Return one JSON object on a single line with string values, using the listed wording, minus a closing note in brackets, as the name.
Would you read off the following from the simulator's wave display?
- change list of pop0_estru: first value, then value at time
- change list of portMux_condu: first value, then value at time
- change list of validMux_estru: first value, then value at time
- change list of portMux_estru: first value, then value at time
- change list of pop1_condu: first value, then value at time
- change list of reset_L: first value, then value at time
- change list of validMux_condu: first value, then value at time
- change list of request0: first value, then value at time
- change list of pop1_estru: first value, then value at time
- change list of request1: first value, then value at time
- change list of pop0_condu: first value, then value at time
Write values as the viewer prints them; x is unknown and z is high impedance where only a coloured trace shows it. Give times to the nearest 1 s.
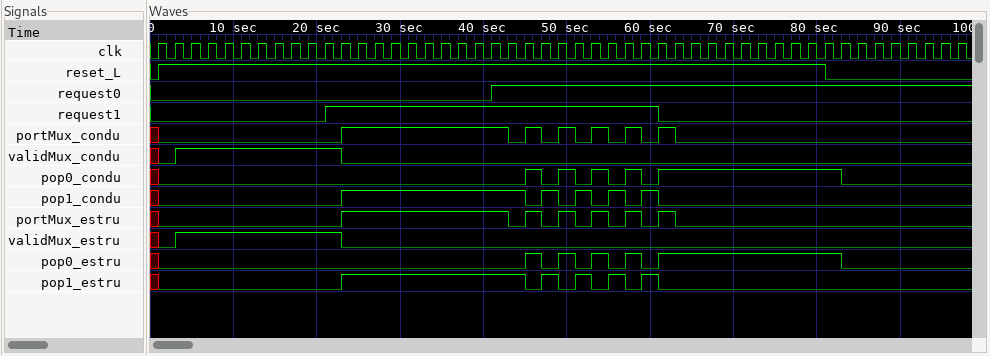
{"change list of pop0_estru: first value, then value at time": "x, 0 at 1 s, 1 at 45 s, 0 at 47 s, 1 at 49 s, 0 at 51 s, 1 at 53 s, 0 at 55 s, 1 at 57 s, 0 at 59 s, 1 at 61 s, 0 at 83 s", "change list of portMux_condu: first value, then value at time": "x, 0 at 1 s, 1 at 23 s, 0 at 43 s, 1 at 45 s, 0 at 47 s, 1 at 49 s, 0 at 51 s, 1 at 53 s, 0 at 55 s, 1 at 57 s, 0 at 59 s, 1 at 61 s, 0 at 63 s", "change list of validMux_estru: first value, then value at time": "x, 0 at 1 s, 1 at 3 s, 0 at 23 s", "change list of portMux_estru: first value, then value at time": "x, 0 at 1 s, 1 at 23 s, 0 at 43 s, 1 at 45 s, 0 at 47 s, 1 at 49 s, 0 at 51 s, 1 at 53 s, 0 at 55 s, 1 at 57 s, 0 at 59 s, 1 at 61 s, 0 at 63 s", "change list of pop1_condu: first value, then value at time": "x, 0 at 1 s, 1 at 23 s, 0 at 45 s, 1 at 47 s, 0 at 49 s, 1 at 51 s, 0 at 53 s, 1 at 55 s, 0 at 57 s, 1 at 59 s, 0 at 61 s", "change list of reset_L: first value, then value at time": "0, 1 at 1 s, 0 at 81 s", "change list of validMux_condu: first value, then value at time": "x, 0 at 1 s, 1 at 3 s, 0 at 23 s", "change list of request0: first value, then value at time": "0, 1 at 41 s", "change list of pop1_estru: first value, then value at time": "x, 0 at 1 s, 1 at 23 s, 0 at 45 s, 1 at 47 s, 0 at 49 s, 1 at 51 s, 0 at 53 s, 1 at 55 s, 0 at 57 s, 1 at 59 s, 0 at 61 s", "change list of request1: first value, then value at time": "0, 1 at 21 s, 0 at 61 s", "change list of pop0_condu: first value, then value at time": "x, 0 at 1 s, 1 at 45 s, 0 at 47 s, 1 at 49 s, 0 at 51 s, 1 at 53 s, 0 at 55 s, 1 at 57 s, 0 at 59 s, 1 at 61 s, 0 at 83 s"}
